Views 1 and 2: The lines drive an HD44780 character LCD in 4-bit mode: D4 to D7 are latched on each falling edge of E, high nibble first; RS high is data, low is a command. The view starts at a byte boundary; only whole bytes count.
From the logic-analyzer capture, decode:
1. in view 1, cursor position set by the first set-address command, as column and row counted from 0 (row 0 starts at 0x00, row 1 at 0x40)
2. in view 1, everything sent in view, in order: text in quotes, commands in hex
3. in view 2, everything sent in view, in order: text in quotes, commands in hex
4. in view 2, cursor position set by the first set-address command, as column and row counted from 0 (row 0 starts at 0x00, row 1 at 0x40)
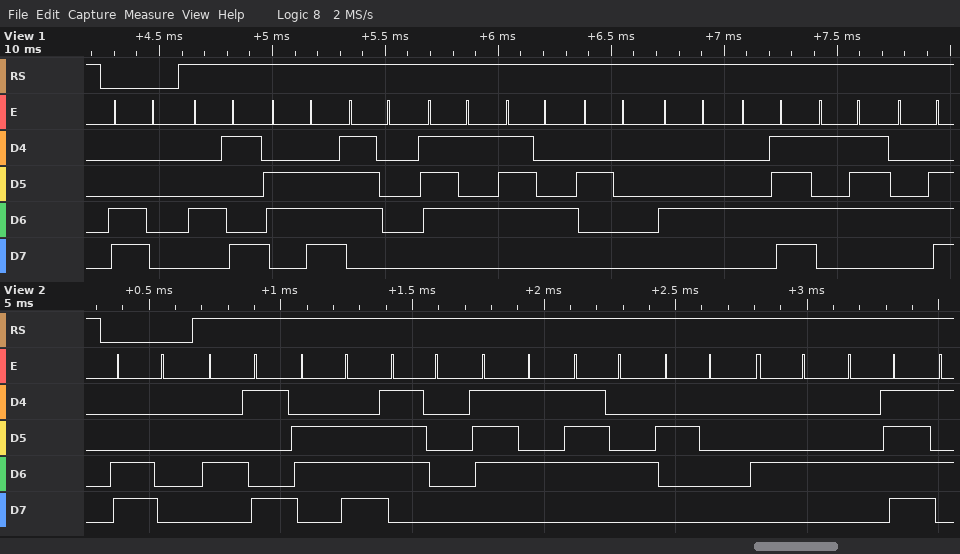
column 0, row 1
0xC0 "Input DOWN"
0xC0 "Input DO"
column 0, row 1
